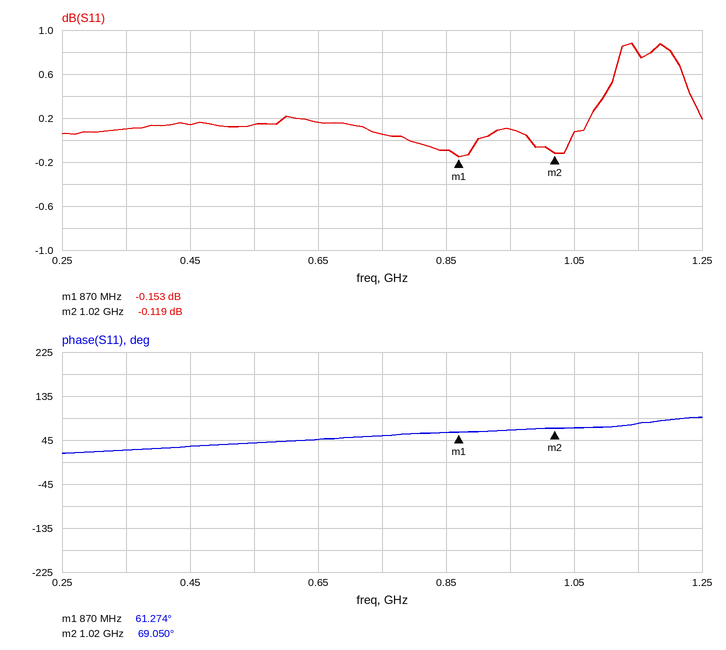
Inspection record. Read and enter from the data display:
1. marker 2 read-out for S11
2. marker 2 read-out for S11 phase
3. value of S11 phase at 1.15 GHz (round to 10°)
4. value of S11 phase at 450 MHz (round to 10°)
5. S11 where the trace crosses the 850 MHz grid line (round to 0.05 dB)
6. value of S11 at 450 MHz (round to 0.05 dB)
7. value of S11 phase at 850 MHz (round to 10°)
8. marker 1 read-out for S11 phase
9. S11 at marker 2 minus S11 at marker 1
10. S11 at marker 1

-0.119 dB
69.050°
80°
30°
-0.10 dB
0.15 dB
60°
61.274°
0.034 dB
-0.153 dB
